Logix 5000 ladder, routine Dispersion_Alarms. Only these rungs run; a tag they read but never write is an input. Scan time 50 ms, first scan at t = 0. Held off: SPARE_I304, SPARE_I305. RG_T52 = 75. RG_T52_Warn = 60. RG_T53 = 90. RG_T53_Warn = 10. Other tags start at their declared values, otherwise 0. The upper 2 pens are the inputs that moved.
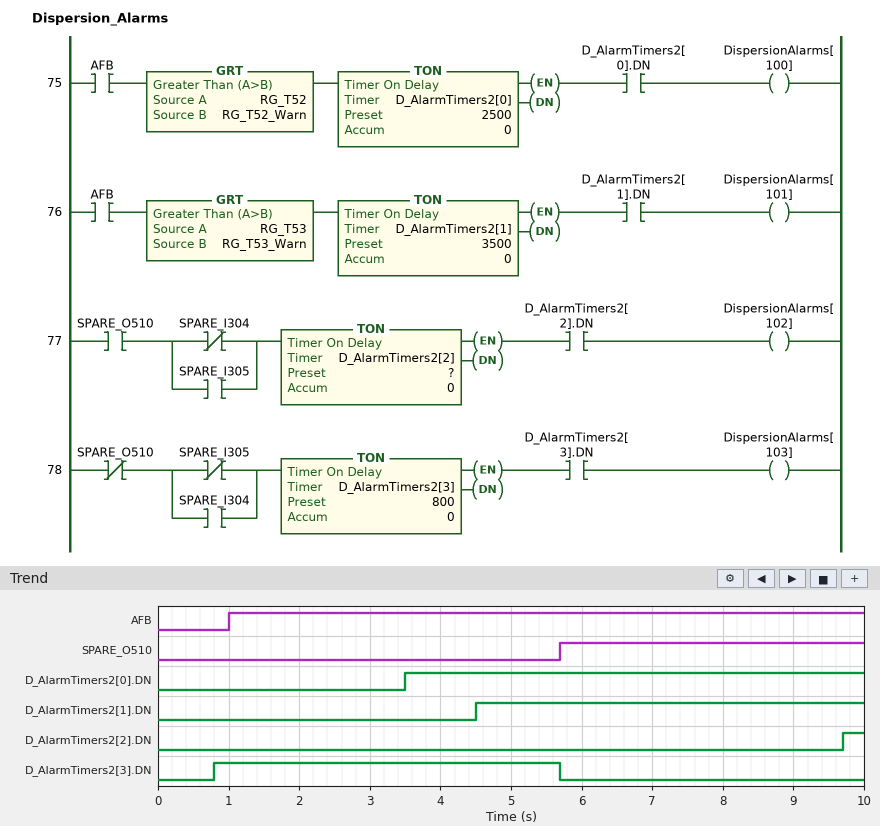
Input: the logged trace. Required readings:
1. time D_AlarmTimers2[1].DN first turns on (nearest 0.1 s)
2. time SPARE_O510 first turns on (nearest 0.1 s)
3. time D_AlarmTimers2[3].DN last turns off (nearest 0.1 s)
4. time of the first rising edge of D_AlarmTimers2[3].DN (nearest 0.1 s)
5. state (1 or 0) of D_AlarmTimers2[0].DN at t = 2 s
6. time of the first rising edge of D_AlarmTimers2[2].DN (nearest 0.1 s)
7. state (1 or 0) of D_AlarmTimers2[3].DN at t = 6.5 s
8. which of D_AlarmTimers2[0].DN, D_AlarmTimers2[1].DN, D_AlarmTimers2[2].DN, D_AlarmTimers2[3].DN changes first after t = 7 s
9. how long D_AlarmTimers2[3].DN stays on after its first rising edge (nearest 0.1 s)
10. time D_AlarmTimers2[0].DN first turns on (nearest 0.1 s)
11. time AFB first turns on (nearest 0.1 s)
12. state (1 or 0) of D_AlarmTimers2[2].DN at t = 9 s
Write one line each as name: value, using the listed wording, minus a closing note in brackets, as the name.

time D_AlarmTimers2[1].DN first turns on: 4.5 s
time SPARE_O510 first turns on: 5.7 s
time D_AlarmTimers2[3].DN last turns off: 5.7 s
time of the first rising edge of D_AlarmTimers2[3].DN: 0.8 s
state (1 or 0) of D_AlarmTimers2[0].DN at t = 2 s: 0
time of the first rising edge of D_AlarmTimers2[2].DN: 9.7 s
state (1 or 0) of D_AlarmTimers2[3].DN at t = 6.5 s: 0
which of D_AlarmTimers2[0].DN, D_AlarmTimers2[1].DN, D_AlarmTimers2[2].DN, D_AlarmTimers2[3].DN changes first after t = 7 s: D_AlarmTimers2[2].DN
how long D_AlarmTimers2[3].DN stays on after its first rising edge: 4.9 s
time D_AlarmTimers2[0].DN first turns on: 3.5 s
time AFB first turns on: 1.0 s
state (1 or 0) of D_AlarmTimers2[2].DN at t = 9 s: 0
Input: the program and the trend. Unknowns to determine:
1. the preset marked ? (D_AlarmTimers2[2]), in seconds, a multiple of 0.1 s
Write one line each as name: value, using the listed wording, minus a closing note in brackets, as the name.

the preset marked ? (D_AlarmTimers2[2]), in seconds, a multiple of 0.1 s: 4.0 s
